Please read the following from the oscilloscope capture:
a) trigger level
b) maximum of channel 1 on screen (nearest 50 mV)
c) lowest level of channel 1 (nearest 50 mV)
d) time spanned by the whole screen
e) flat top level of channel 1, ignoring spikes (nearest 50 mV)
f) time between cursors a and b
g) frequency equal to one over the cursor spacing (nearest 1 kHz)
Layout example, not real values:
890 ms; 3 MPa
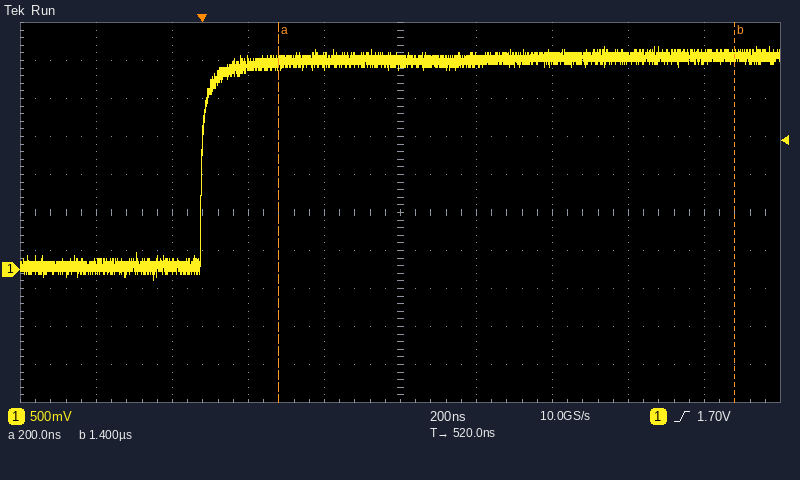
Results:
1.70 V; 2.95 V; -150 mV; 2 µs; 2.80 V; 1.20 µs; 833 kHz
